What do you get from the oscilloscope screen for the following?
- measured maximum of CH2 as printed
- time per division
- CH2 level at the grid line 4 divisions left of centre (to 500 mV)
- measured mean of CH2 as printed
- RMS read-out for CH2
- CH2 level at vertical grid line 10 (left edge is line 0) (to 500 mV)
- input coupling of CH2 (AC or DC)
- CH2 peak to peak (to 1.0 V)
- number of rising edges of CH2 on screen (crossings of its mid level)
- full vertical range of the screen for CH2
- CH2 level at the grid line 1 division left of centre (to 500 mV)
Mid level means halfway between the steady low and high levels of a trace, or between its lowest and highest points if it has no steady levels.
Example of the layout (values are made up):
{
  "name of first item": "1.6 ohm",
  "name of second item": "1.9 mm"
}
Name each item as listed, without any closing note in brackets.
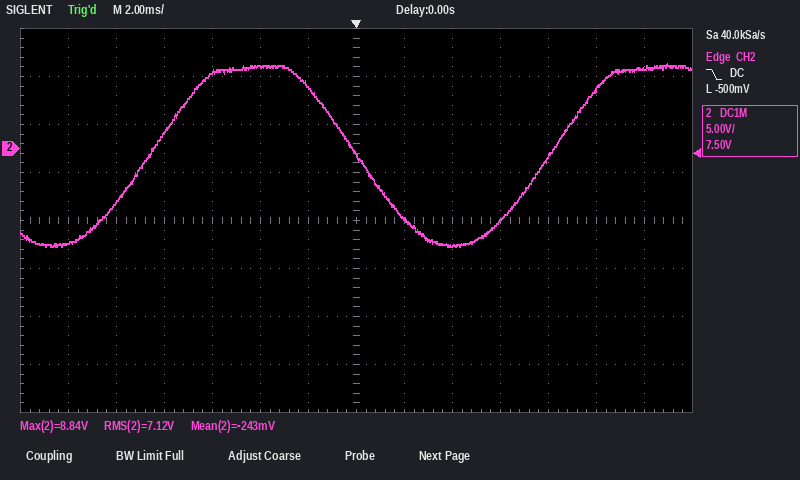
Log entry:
{
  "measured maximum of CH2 as printed": "8.84 V",
  "time per division": "2 ms",
  "CH2 level at the grid line 4 divisions left of centre": "1.5 V",
  "measured mean of CH2 as printed": "-243 mV",
  "RMS read-out for CH2": "7.12 V",
  "CH2 level at vertical grid line 10 (left edge is line 0)": "-7.5 V",
  "input coupling of CH2": "DC",
  "CH2 peak to peak": "19.0 V",
  "number of rising edges of CH2 on screen": "2",
  "full vertical range of the screen for CH2": "40 V",
  "CH2 level at the grid line 1 division left of centre": "6.5 V"
}
